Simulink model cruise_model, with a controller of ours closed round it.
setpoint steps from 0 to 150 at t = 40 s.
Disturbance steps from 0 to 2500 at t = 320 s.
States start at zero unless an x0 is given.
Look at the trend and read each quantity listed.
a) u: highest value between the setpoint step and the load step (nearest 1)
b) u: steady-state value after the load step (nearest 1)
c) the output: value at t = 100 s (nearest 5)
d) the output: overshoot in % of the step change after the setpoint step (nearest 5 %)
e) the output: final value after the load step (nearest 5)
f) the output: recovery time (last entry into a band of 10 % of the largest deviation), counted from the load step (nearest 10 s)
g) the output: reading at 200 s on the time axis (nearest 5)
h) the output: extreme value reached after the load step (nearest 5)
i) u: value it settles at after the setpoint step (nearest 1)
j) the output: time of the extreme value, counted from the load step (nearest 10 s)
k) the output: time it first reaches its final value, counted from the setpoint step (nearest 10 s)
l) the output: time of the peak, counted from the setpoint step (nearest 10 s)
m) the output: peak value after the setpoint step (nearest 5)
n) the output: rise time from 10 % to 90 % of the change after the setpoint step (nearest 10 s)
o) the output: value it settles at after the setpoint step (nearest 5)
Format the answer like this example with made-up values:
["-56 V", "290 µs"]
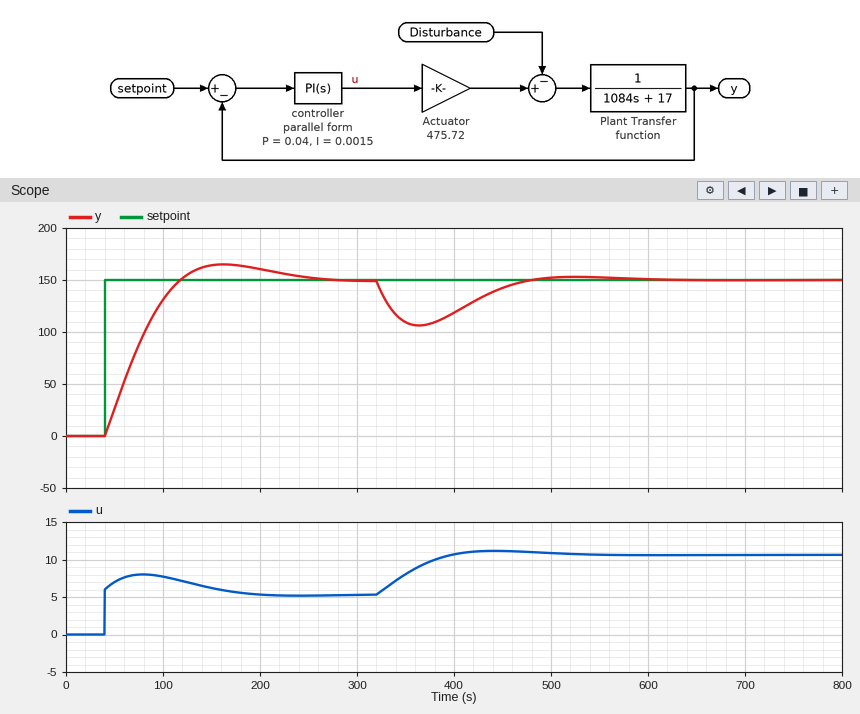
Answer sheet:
["8", "11", "130", "10 %", "150", "140 s", "160", "105", "5", "40 s", "80 s", "120 s", "165", "60 s", "150"]
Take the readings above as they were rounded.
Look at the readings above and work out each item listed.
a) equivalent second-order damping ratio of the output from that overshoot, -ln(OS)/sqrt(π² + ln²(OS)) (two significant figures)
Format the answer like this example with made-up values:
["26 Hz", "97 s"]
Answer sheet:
["0.59"]
